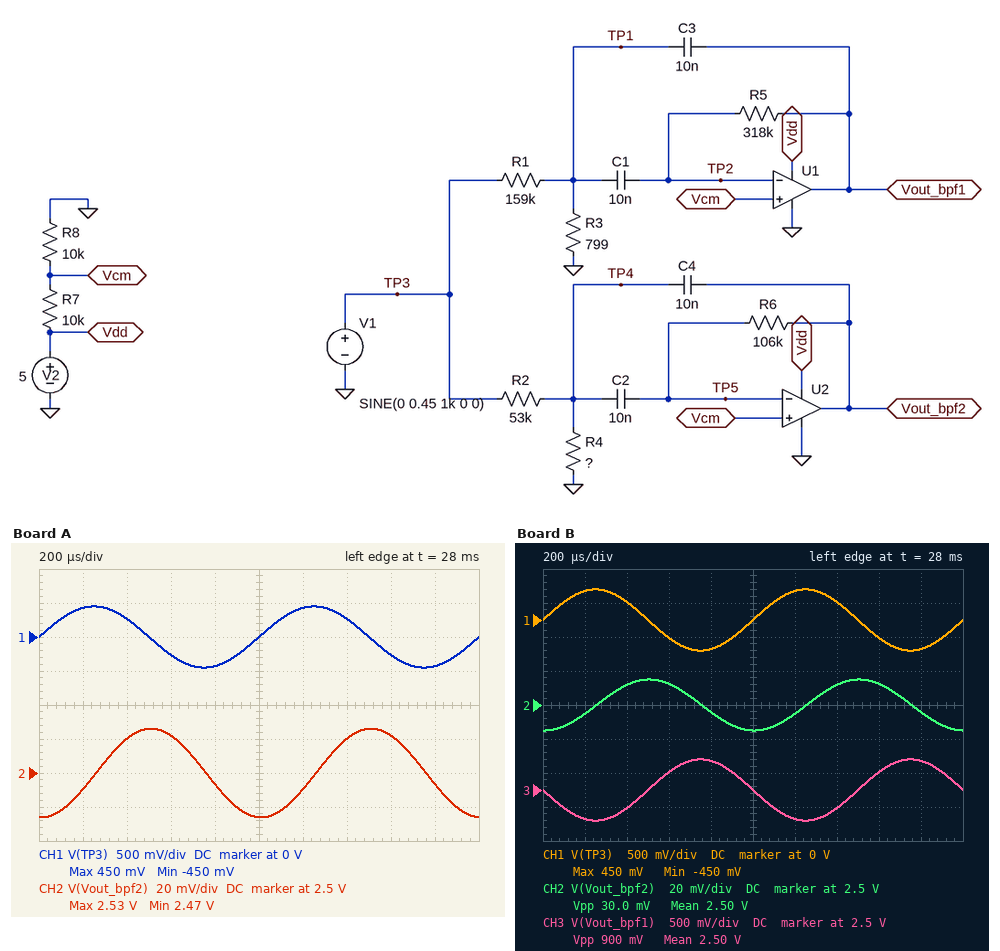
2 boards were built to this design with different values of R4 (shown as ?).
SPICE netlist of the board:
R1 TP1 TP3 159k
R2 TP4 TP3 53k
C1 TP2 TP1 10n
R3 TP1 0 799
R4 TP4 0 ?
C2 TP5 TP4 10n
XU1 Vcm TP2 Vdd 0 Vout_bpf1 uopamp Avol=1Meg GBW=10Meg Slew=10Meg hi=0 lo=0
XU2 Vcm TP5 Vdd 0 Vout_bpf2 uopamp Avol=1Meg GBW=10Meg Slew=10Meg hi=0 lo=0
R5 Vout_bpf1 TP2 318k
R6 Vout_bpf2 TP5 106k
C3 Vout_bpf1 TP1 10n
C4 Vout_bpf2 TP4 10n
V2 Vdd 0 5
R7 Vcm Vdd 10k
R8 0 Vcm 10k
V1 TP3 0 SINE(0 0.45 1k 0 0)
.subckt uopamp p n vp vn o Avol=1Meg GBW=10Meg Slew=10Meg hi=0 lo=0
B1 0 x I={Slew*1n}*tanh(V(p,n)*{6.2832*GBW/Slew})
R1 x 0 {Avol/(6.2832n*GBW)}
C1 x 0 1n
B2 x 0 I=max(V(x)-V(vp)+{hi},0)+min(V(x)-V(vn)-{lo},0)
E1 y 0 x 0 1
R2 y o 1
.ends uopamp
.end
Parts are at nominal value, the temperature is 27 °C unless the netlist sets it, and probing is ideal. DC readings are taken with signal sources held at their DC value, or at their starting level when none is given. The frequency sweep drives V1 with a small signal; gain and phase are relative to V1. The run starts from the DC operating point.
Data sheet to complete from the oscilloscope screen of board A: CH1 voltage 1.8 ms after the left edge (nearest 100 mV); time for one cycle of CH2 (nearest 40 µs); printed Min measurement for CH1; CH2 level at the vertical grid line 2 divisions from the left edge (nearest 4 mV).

-400 mV
1.00 ms
-450 mV
2.520 V
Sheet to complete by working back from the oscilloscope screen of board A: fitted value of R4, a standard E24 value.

390 Ω
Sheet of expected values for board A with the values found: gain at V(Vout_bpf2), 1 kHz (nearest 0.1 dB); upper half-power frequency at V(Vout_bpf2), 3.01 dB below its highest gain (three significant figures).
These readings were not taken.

-24.7 dB
2.63 kHz
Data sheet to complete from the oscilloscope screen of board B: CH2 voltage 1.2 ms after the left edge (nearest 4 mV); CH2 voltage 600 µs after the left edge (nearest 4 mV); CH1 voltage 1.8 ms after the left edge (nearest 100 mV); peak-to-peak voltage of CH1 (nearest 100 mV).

2.496 V
2.512 V
-400 mV
900 mV
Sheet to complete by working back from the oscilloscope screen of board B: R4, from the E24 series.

240 Ω
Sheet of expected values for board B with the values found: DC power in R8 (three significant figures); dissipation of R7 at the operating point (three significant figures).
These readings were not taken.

625 µW
625 µW
